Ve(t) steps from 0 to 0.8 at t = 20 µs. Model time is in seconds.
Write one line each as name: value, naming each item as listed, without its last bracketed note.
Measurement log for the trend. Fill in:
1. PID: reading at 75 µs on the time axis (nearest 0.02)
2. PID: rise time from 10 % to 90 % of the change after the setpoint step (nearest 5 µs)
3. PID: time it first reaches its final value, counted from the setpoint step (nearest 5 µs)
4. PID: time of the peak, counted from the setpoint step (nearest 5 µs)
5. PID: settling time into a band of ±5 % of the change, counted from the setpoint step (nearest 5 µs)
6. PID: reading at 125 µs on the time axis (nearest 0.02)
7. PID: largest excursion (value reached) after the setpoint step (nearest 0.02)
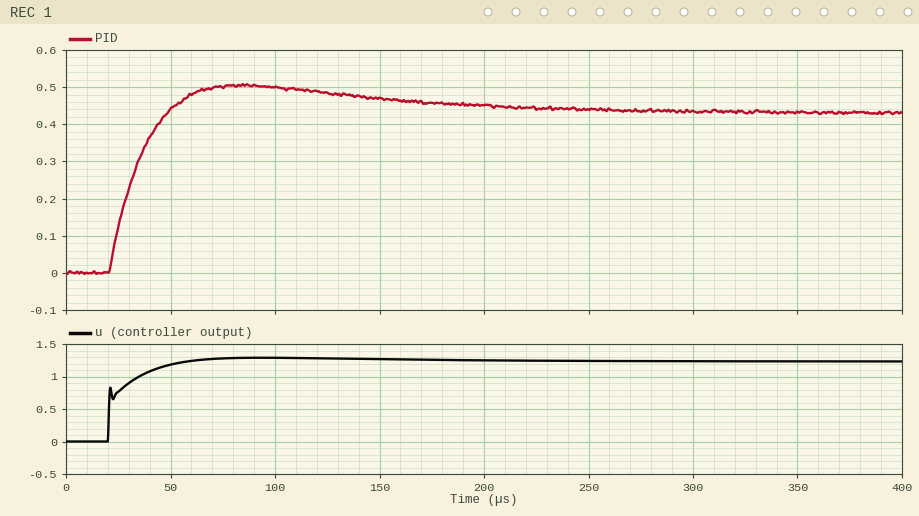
PID: reading at 75 µs on the time axis: 0.50
PID: rise time from 10 % to 90 % of the change after the setpoint step: 20 µs
PID: time it first reaches its final value, counted from the setpoint step: 30 µs
PID: time of the peak, counted from the setpoint step: 65 µs
PID: settling time into a band of ±5 % of the change, counted from the setpoint step: 175 µs
PID: reading at 125 µs on the time axis: 0.48
PID: largest excursion (value reached) after the setpoint step: 0.50
